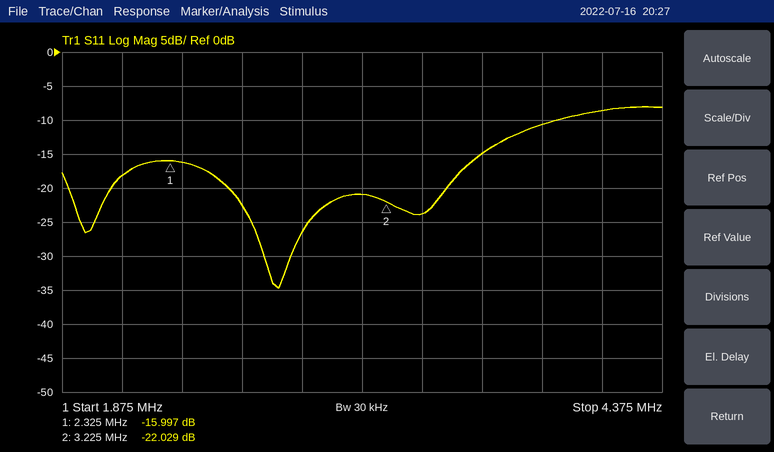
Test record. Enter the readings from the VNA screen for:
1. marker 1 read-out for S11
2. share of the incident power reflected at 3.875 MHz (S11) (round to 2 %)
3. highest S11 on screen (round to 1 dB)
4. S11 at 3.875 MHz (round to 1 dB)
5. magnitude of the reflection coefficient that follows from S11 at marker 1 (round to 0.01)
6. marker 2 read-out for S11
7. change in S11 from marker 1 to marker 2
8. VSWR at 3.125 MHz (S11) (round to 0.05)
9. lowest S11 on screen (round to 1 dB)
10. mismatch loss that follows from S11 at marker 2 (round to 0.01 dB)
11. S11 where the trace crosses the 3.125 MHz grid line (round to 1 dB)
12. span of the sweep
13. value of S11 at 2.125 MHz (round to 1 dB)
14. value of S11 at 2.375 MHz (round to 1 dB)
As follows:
-15.997 dB
8 %
-8 dB
-11 dB
0.16
-22.029 dB
-6.032 dB
1.20
-35 dB
0.03 dB
-21 dB
2.5 MHz
-18 dB
-16 dB
